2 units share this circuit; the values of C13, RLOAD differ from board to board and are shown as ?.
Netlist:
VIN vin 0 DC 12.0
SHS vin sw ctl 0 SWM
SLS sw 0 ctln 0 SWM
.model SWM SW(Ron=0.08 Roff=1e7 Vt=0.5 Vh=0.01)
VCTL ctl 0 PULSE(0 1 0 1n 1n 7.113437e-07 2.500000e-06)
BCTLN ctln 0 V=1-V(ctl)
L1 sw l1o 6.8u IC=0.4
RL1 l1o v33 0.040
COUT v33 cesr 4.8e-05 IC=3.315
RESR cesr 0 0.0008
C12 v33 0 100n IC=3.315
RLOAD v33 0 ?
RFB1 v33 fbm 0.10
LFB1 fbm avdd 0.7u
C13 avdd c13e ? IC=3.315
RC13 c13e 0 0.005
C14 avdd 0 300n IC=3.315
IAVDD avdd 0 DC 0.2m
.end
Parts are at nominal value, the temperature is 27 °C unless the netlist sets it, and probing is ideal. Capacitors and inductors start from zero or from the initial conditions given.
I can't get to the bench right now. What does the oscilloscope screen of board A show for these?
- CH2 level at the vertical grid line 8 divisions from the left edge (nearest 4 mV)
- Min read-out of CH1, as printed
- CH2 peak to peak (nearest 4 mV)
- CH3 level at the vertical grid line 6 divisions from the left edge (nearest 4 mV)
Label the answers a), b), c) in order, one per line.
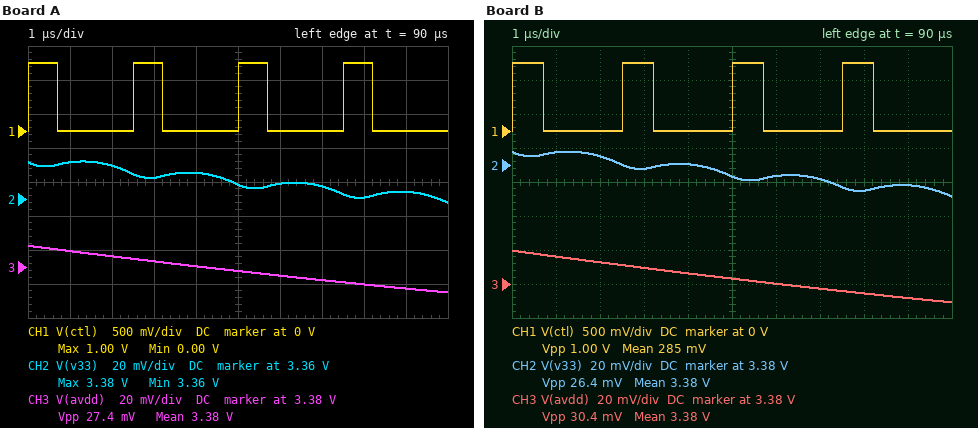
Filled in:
a) 3.360 V
b) 0.00 V
c) 24 mV
d) 3.376 V
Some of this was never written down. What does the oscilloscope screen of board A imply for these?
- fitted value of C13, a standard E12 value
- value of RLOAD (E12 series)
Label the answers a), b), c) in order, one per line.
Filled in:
a) 33 µF
b) 18 Ω
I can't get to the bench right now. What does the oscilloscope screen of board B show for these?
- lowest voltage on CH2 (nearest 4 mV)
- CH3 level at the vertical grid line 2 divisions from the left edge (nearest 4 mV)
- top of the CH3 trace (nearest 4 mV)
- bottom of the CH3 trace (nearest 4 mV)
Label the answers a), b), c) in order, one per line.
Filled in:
a) 3.360 V
b) 3.392 V
c) 3.400 V
d) 3.368 V
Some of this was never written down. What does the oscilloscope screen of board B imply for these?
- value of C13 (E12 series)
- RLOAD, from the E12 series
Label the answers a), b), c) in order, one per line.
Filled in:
a) 33 µF
b) 27 Ω
